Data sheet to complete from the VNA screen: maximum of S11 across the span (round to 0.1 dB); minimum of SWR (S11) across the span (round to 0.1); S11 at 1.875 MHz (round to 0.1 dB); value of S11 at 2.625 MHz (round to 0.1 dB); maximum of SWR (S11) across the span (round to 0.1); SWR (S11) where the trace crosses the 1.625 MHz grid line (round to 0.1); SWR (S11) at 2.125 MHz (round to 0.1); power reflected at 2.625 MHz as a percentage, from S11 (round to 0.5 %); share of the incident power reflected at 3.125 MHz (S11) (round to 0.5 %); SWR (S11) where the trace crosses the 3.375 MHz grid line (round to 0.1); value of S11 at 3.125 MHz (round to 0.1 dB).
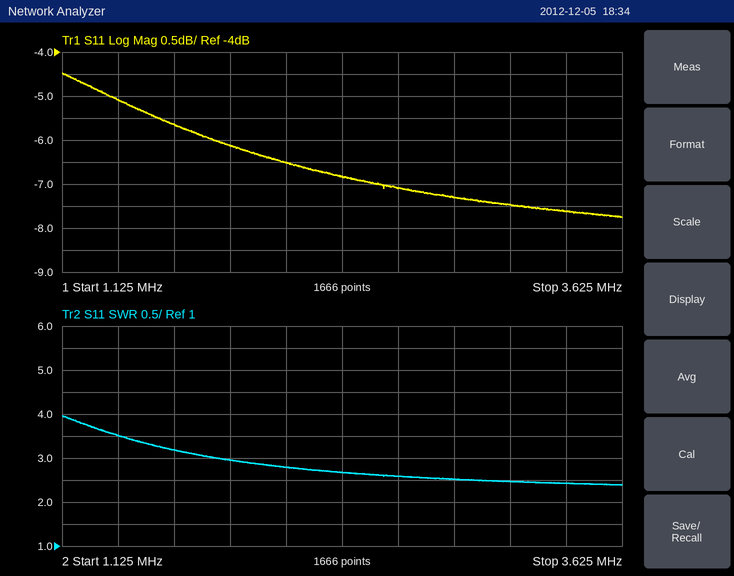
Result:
-4.5 dB
2.4
-6.1 dB
-7.1 dB
4.0
3.2
2.8
19.5 %
18.0 %
2.4
-7.5 dB
